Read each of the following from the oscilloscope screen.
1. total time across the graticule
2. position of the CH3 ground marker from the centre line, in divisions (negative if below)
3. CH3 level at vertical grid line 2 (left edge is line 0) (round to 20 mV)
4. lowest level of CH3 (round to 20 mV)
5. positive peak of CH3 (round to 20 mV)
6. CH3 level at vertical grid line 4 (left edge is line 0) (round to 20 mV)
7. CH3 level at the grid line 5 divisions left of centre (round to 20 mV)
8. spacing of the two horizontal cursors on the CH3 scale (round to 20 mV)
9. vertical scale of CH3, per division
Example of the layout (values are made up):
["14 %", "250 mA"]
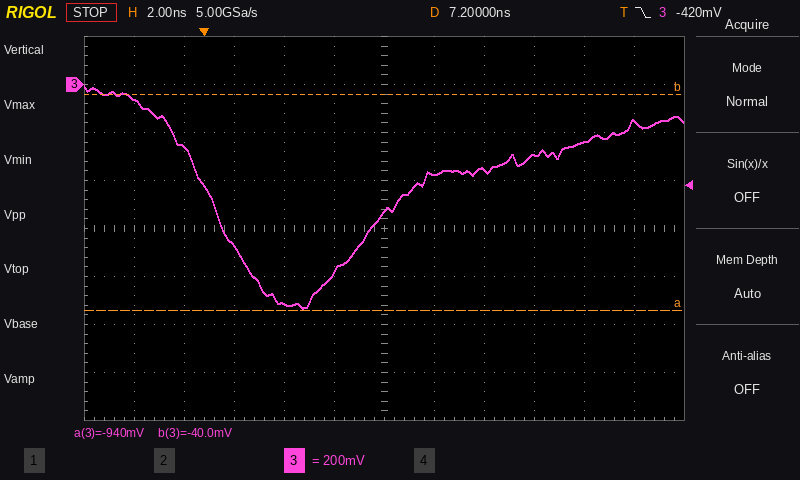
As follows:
["24 ns", "+3.0 div", "-260 mV", "-940 mV", "0 mV", "-920 mV", "-60 mV", "900 mV", "200 mV"]
